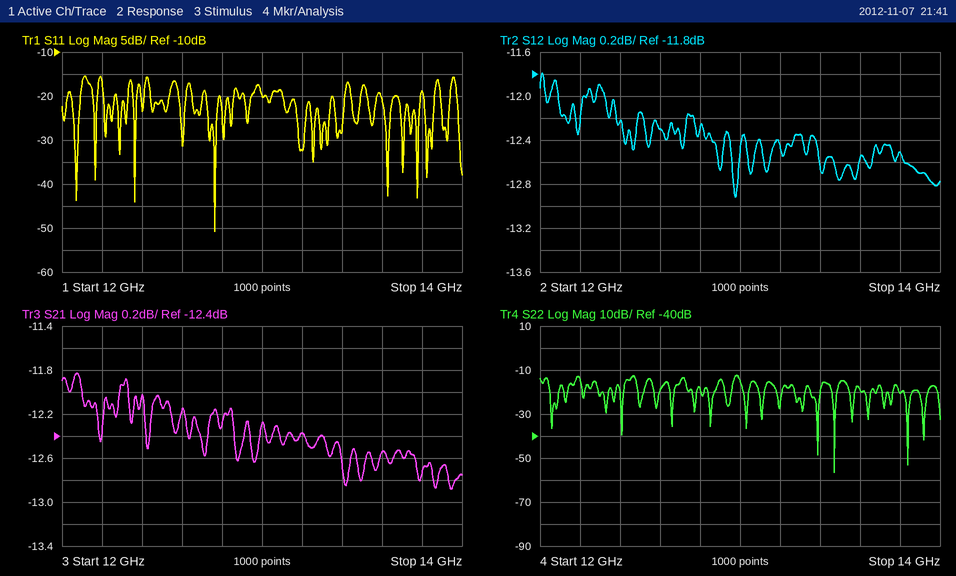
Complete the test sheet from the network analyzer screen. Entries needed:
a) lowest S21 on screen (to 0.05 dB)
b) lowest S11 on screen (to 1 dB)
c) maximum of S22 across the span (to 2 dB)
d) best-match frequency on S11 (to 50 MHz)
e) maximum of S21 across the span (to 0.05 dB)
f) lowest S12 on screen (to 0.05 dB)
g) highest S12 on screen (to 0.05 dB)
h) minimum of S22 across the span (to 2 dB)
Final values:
-12.90 dB
-51 dB
-12 dB
12.75 GHz
-11.85 dB
-12.90 dB
-11.80 dB
-56 dB
